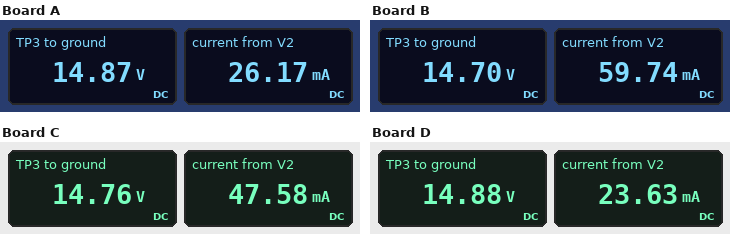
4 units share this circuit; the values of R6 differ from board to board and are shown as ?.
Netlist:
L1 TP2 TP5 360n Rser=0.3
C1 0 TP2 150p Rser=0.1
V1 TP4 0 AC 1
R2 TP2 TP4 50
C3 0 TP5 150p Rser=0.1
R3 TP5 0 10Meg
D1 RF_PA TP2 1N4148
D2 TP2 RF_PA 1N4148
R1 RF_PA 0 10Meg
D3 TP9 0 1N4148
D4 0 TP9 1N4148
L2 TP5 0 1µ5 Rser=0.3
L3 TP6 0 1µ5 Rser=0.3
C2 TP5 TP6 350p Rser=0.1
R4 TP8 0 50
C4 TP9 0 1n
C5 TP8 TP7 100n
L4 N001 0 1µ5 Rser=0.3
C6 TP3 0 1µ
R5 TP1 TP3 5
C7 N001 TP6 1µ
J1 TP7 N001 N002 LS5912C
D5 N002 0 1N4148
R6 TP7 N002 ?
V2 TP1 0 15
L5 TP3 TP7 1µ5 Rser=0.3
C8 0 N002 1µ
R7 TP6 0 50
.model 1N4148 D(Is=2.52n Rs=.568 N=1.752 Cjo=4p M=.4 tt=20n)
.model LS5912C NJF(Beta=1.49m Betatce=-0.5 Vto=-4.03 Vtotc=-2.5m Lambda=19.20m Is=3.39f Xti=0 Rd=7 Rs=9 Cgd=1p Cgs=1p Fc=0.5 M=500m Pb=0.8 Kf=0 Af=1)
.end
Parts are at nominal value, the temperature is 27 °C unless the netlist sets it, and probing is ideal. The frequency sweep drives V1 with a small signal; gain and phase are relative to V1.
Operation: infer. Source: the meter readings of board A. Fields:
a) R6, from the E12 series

1.8 kΩ
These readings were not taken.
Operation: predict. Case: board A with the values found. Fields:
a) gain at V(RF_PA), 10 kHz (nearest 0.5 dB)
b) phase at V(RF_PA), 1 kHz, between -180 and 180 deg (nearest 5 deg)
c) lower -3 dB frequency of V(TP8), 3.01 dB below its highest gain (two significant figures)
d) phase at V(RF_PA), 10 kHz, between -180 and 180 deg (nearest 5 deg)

-39.0 dB
10 deg
7.3 MHz
20 deg
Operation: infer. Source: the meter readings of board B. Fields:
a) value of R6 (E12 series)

330 Ω
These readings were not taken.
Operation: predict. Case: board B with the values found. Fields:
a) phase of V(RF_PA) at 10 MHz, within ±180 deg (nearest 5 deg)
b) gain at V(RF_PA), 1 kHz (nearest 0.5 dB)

-5 deg
-43.5 dB
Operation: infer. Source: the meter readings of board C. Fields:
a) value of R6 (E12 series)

470 Ω
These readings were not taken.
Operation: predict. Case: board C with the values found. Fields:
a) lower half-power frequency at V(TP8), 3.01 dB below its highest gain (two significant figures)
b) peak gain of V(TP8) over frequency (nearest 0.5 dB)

7.2 MHz
-13.0 dB
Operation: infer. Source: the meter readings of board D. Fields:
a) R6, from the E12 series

2.7 kΩ
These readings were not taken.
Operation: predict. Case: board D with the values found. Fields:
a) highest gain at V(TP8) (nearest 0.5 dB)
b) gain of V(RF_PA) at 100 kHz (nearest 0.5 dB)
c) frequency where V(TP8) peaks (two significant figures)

-12.0 dB
-31.5 dB
21 MHz
